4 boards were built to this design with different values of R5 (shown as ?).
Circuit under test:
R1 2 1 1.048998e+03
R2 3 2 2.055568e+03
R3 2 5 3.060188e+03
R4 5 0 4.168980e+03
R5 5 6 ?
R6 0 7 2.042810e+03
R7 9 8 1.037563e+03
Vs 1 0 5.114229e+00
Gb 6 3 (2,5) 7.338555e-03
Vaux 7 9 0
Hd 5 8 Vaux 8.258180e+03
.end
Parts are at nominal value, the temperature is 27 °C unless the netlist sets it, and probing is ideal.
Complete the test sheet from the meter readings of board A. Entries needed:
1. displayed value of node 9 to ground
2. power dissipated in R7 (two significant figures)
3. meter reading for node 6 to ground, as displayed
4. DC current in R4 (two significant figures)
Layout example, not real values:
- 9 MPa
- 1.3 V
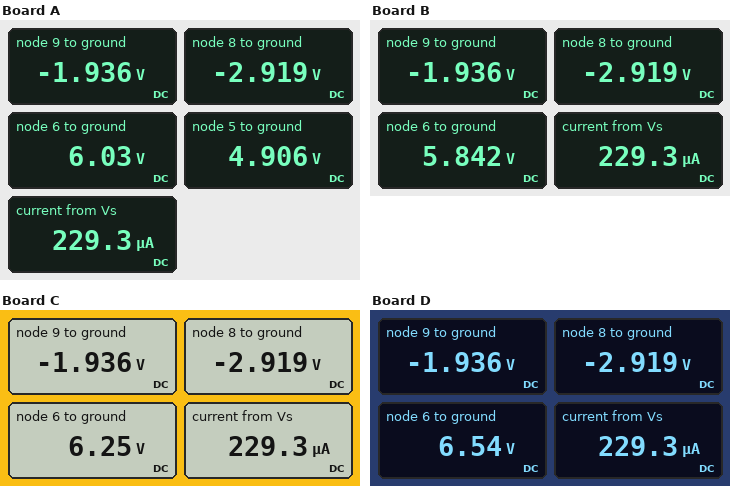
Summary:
- -1.936 V
- 930 µW
- 6.03 V
- 1.2 mA
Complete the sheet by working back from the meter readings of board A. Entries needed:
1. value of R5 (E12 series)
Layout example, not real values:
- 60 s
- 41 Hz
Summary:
- 4.7 kΩ
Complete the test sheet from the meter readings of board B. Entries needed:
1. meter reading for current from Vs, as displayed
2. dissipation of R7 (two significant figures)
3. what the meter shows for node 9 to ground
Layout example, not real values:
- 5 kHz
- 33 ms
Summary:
- 229.3 µA
- 930 µW
- -1.936 V
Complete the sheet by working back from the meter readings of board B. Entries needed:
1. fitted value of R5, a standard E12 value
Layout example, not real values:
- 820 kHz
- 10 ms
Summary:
- 3.9 kΩ
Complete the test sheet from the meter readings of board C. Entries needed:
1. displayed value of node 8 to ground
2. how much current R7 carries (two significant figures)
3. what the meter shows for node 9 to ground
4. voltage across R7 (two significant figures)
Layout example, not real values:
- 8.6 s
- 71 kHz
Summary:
- -2.919 V
- 950 µA
- -1.936 V
- 980 mV
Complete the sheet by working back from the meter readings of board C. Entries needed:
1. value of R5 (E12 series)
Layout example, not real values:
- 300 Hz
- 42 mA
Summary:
- 5.6 kΩ
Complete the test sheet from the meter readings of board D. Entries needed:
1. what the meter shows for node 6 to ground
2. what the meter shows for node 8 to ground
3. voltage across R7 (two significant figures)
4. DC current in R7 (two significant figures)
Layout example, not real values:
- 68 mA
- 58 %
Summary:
- 6.54 V
- -2.919 V
- 980 mV
- 950 µA
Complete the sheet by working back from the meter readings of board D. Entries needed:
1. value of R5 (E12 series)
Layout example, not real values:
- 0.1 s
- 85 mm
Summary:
- 6.8 kΩ
